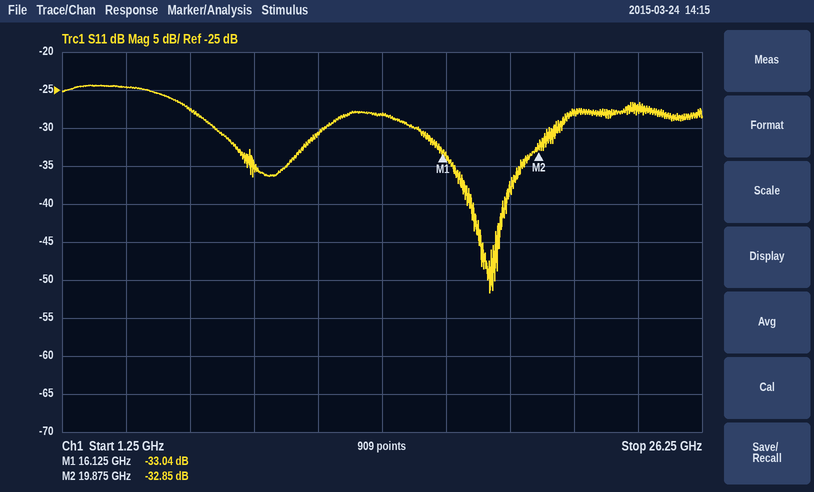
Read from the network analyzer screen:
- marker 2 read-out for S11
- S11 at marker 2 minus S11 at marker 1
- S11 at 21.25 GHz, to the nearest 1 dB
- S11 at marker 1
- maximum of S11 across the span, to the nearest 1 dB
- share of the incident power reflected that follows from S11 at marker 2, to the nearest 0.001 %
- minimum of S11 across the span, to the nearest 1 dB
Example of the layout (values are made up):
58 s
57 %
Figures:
-32.85 dB
0.19 dB
-28 dB
-33.04 dB
-24 dB
0.052 %
-52 dB
